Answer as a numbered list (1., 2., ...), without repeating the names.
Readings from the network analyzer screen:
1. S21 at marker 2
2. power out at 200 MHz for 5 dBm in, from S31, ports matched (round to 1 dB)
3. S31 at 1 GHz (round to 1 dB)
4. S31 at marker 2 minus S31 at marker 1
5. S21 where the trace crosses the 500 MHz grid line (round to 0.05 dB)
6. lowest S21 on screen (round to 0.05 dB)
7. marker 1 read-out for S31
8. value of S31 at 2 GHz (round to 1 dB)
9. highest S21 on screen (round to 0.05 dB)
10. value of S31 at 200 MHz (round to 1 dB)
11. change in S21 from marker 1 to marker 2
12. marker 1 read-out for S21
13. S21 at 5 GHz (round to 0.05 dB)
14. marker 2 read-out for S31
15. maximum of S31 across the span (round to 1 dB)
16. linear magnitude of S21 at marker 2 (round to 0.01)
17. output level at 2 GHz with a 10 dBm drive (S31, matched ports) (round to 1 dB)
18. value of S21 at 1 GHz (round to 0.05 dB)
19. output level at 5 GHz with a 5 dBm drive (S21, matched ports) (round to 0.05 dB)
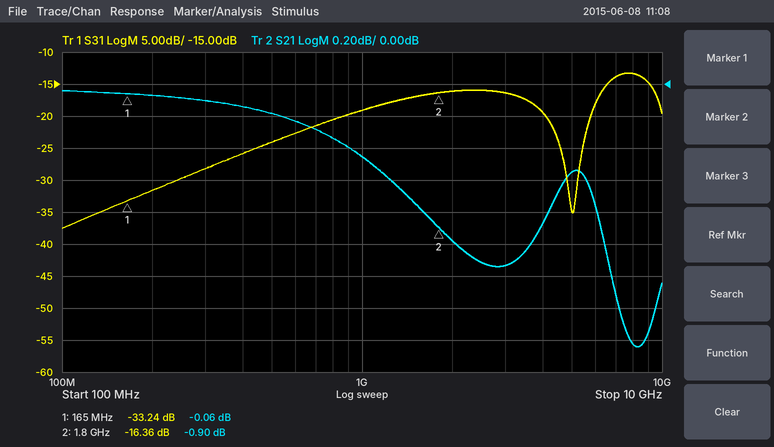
1. -0.90 dB
2. -27 dBm
3. -19 dB
4. 16.88 dB
5. -0.20 dB
6. -1.65 dB
7. -33.24 dB
8. -16 dB
9. -0.05 dB
10. -32 dB
11. -0.84 dB
12. -0.06 dB
13. -0.55 dB
14. -16.36 dB
15. -13 dB
16. 0.90
17. -6 dBm
18. -0.45 dB
19. 4.45 dBm
